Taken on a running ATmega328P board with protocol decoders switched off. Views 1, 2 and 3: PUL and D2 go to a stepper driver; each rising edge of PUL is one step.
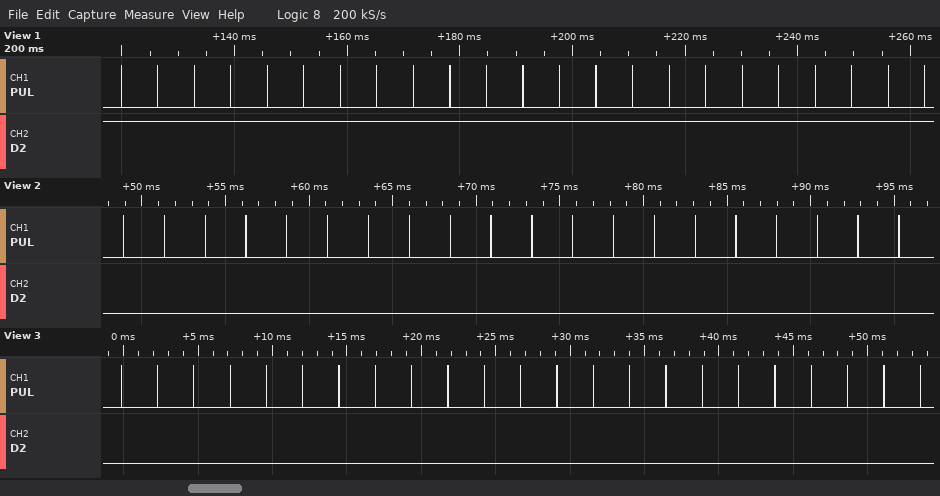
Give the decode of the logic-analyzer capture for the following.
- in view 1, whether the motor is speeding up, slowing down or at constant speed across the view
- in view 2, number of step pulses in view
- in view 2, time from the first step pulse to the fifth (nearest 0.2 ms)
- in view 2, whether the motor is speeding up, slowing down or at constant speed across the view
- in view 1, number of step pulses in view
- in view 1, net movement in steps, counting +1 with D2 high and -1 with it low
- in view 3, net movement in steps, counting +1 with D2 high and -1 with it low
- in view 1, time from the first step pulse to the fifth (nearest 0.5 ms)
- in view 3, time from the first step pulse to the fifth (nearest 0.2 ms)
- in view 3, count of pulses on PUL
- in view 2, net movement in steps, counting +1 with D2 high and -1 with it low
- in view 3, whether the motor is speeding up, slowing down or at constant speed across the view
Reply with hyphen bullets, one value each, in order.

- constant speed
- 20
- 9.8 ms
- constant speed
- 23
- +23
- -23
- 26.0 ms
- 9.8 ms
- 23
- -20
- constant speed
